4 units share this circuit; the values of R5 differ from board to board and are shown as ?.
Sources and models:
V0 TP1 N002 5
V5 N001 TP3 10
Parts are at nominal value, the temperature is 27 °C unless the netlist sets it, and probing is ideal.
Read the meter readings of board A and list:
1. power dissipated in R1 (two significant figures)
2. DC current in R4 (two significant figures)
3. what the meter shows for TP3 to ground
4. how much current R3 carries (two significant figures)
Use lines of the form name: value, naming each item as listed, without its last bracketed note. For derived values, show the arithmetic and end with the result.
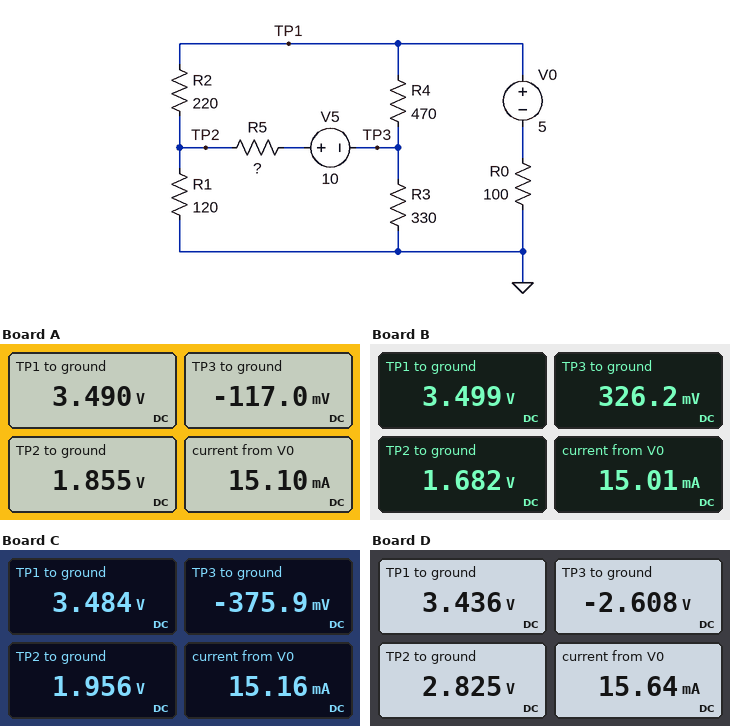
power dissipated in R1: (1.855 V)^2 / 120 Ω = 29 mW
DC current in R4: (3.49 V - (-117 mV)) / 470 Ω = 7.7 mA
what the meter shows for TP3 to ground: -117.0 mV
how much current R3 carries: (0 V - (-117 mV)) / 330 Ω = 350 µA
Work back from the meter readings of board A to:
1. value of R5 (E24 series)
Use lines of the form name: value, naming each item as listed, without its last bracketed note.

value of R5: 1 kΩ
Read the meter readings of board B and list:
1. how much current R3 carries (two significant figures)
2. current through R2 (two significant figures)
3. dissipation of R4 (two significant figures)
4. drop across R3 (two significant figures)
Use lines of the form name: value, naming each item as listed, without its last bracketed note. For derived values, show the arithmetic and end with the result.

how much current R3 carries: (326.2 mV) / 330 Ω = 990 µA
current through R2: (3.499 V - 1.682 V) / 220 Ω = 8.3 mA
dissipation of R4: (3.499 V - 326.2 mV)^2 / 470 Ω = 21 mW
drop across R3: 326.2 mV = 330 mV
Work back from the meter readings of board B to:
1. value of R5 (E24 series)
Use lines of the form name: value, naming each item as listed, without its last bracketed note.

value of R5: 1.5 kΩ
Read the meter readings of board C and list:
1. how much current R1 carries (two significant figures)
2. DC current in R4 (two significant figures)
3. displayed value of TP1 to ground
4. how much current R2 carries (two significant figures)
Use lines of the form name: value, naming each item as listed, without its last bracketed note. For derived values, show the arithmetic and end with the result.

how much current R1 carries: (1.956 V) / 120 Ω = 16 mA
DC current in R4: (3.484 V - (-375.9 mV)) / 470 Ω = 8.2 mA
displayed value of TP1 to ground: 3.484 V
how much current R2 carries: (3.484 V - 1.956 V) / 220 Ω = 6.9 mA
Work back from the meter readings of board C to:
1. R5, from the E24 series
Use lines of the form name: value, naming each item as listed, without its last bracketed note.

R5, from the E24 series: 820 Ω
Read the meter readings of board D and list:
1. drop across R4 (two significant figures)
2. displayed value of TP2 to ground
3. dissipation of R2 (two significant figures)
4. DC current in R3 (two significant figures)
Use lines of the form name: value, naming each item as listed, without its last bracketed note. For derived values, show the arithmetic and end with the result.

drop across R4: 3.436 V - (-2.608 V) = 6.0 V
displayed value of TP2 to ground: 2.825 V
dissipation of R2: (3.436 V - 2.825 V)^2 / 220 Ω = 1.7 mW
DC current in R3: (0 V - (-2.608 V)) / 330 Ω = 7.9 mA
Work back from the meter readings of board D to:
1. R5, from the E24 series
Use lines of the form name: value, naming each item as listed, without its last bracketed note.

R5, from the E24 series: 220 Ω
